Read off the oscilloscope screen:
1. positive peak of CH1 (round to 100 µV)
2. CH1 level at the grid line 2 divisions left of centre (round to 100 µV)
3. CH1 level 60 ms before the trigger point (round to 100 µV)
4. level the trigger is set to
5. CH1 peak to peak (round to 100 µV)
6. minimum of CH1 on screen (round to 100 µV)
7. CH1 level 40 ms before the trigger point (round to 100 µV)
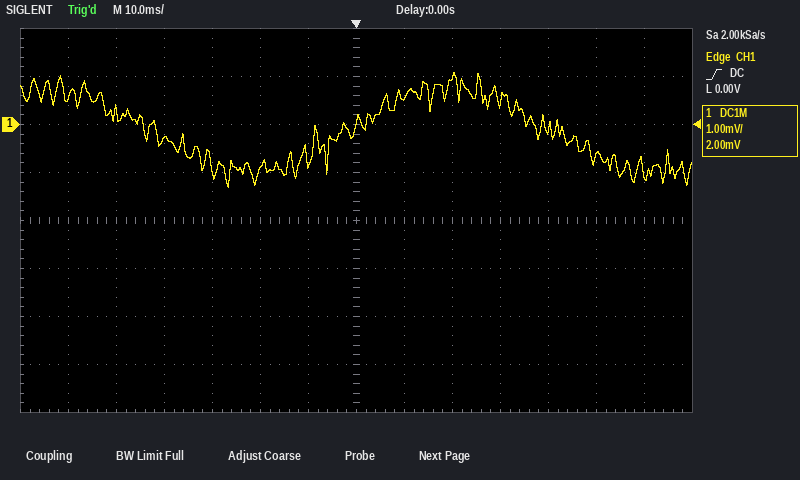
1.1 mV
-900 µV
600 µV
0.00 V
2.4 mV
-1.3 mV
-300 µV
